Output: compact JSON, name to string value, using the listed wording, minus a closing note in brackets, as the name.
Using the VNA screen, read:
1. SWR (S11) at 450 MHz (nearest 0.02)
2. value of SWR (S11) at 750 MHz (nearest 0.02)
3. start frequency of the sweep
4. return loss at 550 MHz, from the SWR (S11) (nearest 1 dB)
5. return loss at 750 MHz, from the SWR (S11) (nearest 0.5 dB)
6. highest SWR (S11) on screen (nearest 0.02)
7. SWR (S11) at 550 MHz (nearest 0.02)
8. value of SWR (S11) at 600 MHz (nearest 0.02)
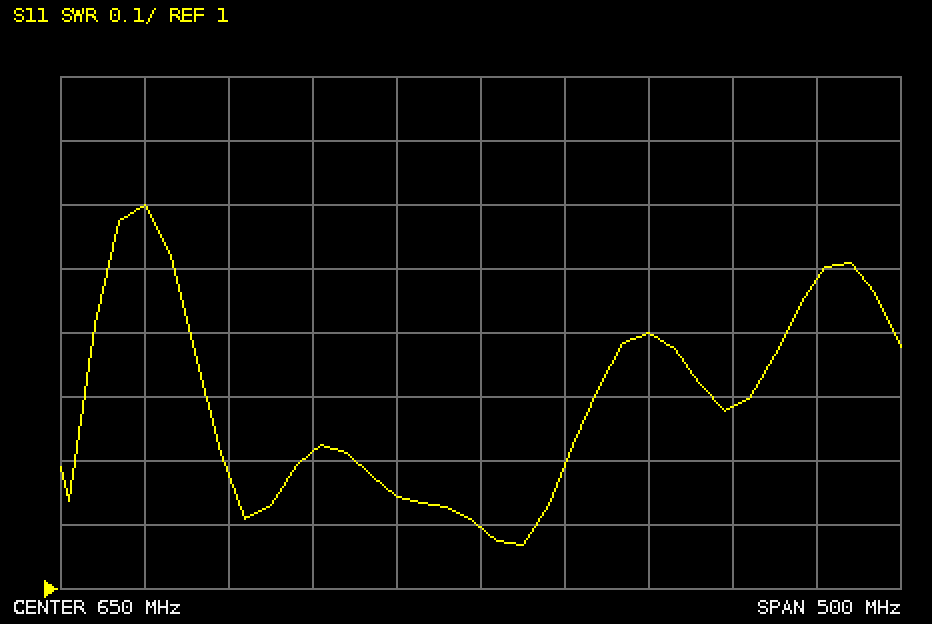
{"SWR (S11) at 450 MHz": "1.60", "value of SWR (S11) at 750 MHz": "1.40", "start frequency of the sweep": "400 MHz", "return loss at 550 MHz, from the SWR (S11)": "20 dB", "return loss at 750 MHz, from the SWR (S11)": "15.5 dB", "highest SWR (S11) on screen": "1.60", "SWR (S11) at 550 MHz": "1.22", "value of SWR (S11) at 600 MHz": "1.14"}
